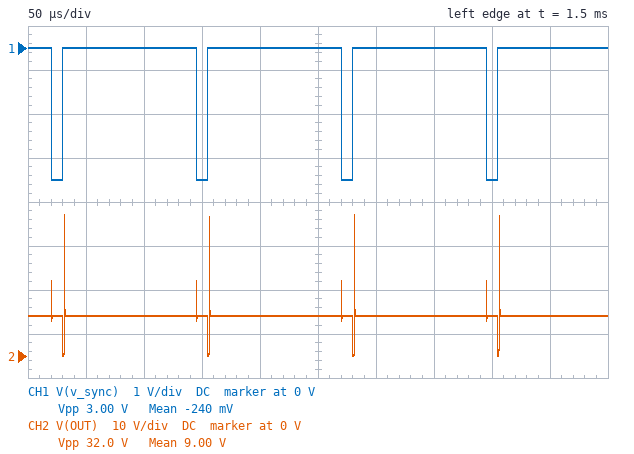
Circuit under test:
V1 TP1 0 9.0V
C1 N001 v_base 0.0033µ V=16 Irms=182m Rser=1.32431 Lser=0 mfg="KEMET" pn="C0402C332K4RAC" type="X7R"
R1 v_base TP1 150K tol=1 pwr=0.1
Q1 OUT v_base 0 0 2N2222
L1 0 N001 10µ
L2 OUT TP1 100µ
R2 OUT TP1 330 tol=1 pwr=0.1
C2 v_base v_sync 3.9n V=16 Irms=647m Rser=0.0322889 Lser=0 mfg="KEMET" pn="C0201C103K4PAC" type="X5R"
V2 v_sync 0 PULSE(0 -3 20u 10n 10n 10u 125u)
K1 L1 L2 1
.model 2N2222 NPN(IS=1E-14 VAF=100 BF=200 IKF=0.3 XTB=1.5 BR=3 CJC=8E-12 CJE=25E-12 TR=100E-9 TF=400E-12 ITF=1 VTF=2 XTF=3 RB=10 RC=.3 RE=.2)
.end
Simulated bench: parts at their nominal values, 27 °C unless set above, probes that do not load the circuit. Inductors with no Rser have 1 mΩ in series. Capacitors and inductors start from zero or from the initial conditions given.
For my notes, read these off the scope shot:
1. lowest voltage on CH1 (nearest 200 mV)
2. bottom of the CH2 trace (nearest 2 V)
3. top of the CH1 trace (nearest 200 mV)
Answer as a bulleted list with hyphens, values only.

- -3.0 V
- 0 V
- 0 V
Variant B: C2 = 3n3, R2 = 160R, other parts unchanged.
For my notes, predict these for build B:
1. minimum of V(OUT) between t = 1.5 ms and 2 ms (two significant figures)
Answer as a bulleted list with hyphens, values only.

- 70 mV
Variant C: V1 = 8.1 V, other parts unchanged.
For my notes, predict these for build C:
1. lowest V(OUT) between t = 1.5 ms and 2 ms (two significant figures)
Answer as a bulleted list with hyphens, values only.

- 45 mV
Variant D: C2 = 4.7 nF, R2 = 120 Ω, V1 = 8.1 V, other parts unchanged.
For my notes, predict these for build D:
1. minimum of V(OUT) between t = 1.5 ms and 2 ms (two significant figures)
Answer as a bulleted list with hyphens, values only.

- 80 mV
